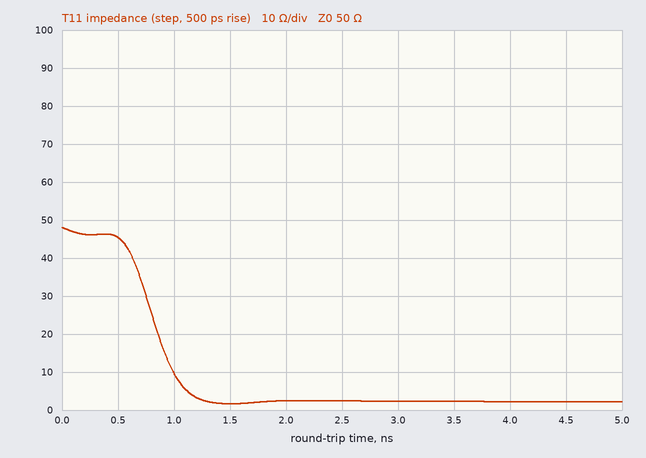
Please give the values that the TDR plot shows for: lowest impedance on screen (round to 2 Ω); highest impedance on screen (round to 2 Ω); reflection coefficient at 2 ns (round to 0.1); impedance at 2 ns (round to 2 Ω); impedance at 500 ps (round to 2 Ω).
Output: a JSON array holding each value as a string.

["2 Ω", "48 Ω", "-0.9", "2 Ω", "46 Ω"]
